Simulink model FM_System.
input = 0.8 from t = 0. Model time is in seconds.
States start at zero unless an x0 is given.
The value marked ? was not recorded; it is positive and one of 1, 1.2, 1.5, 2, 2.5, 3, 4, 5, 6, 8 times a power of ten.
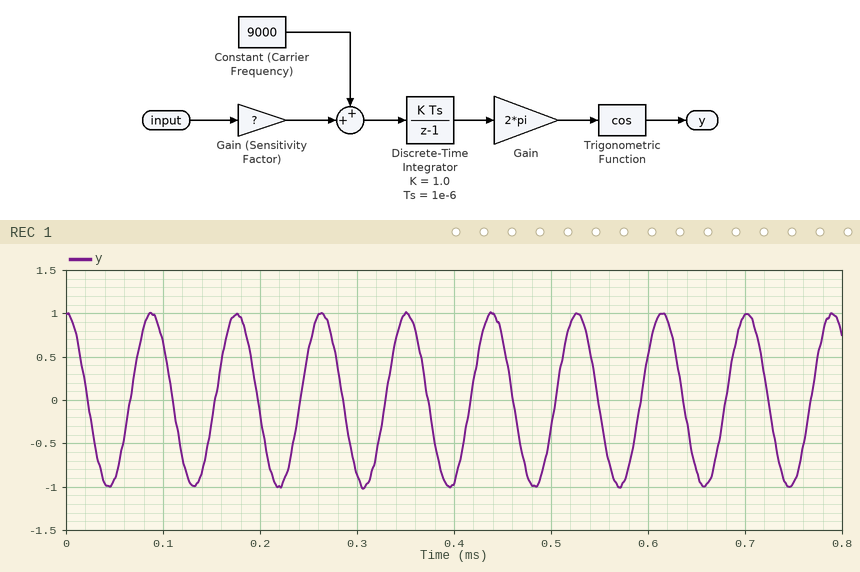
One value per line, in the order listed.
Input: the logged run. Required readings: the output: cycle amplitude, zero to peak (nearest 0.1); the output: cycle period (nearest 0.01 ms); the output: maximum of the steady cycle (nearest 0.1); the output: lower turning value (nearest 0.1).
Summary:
1.0
0.09 ms
1.0
-1.0
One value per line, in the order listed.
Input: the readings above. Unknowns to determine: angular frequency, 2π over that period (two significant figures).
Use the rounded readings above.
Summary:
70 rad/ms
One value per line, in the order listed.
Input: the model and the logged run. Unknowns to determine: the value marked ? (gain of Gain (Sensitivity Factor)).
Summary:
3000
